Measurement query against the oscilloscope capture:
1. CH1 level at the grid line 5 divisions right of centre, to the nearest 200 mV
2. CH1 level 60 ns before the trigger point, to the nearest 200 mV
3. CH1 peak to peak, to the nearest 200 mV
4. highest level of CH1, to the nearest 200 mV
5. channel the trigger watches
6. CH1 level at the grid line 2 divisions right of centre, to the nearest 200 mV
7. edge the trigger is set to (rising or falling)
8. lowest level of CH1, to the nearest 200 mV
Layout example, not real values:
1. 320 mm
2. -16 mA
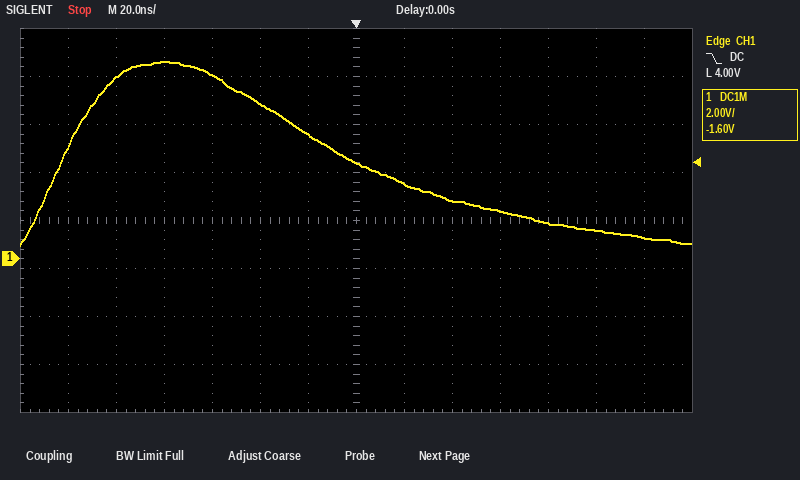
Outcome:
1. 1.2 V
2. 7.6 V
3. 7.6 V
4. 8.2 V
5. CH1
6. 2.4 V
7. falling
8. 600 mV
